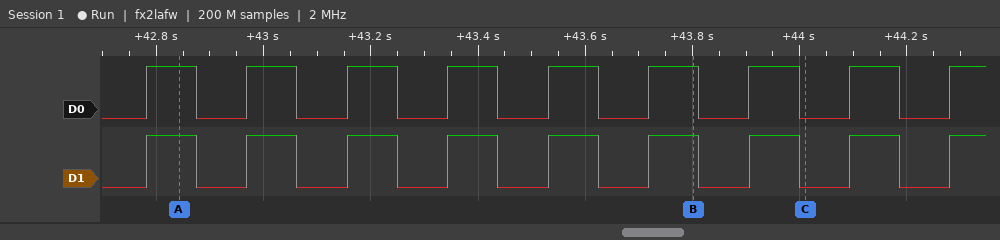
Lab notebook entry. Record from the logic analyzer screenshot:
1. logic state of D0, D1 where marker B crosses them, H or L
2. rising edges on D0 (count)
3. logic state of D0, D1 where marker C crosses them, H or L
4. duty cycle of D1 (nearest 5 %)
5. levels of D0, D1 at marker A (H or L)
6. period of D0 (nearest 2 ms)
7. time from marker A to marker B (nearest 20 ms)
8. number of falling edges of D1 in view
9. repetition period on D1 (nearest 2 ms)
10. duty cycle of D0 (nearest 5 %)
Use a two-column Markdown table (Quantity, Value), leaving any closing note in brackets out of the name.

| Quantity | Value |
|---|---|
| logic state of D0, D1 where marker B crosses them, H or L | D0=H, D1=H |
| rising edges on D0 | 9 |
| logic state of D0, D1 where marker C crosses them, H or L | D0=L, D1=L |
| duty cycle of D1 | 50 % |
| levels of D0, D1 at marker A | D0=H, D1=H |
| period of D0 | 188 ms |
| time from marker A to marker B | 960 ms |
| number of falling edges of D1 in view | 8 |
| repetition period on D1 | 188 ms |
| duty cycle of D0 | 50 % |
